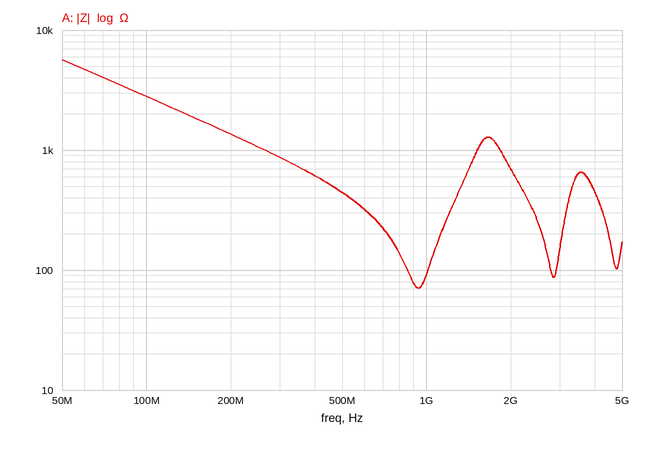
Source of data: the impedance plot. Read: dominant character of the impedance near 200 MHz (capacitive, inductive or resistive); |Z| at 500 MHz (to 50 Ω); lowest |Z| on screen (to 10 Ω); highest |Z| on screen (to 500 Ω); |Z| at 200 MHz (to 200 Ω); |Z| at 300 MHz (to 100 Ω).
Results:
capacitive
450 Ω
70 Ω
5.5 kΩ
1.4 kΩ
900 Ω
